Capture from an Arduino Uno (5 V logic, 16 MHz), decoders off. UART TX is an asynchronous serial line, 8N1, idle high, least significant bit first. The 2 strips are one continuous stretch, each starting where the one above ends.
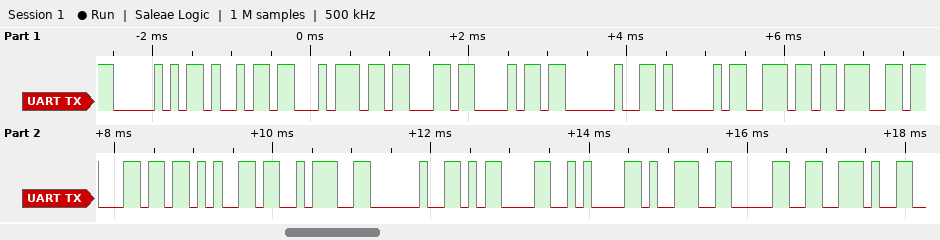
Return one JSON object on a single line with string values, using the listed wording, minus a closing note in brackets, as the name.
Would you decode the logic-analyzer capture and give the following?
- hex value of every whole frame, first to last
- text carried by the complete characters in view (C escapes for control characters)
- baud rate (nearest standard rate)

{"hex value of every whole frame, first to last": "50 69 74 63 68 20 41 6E 67 6C 65 3A 20 0D 0A 39 30 2E", "text carried by the complete characters in view": "\"Pitch Angle: \\r\\n90.\"", "baud rate": "9600 baud"}
